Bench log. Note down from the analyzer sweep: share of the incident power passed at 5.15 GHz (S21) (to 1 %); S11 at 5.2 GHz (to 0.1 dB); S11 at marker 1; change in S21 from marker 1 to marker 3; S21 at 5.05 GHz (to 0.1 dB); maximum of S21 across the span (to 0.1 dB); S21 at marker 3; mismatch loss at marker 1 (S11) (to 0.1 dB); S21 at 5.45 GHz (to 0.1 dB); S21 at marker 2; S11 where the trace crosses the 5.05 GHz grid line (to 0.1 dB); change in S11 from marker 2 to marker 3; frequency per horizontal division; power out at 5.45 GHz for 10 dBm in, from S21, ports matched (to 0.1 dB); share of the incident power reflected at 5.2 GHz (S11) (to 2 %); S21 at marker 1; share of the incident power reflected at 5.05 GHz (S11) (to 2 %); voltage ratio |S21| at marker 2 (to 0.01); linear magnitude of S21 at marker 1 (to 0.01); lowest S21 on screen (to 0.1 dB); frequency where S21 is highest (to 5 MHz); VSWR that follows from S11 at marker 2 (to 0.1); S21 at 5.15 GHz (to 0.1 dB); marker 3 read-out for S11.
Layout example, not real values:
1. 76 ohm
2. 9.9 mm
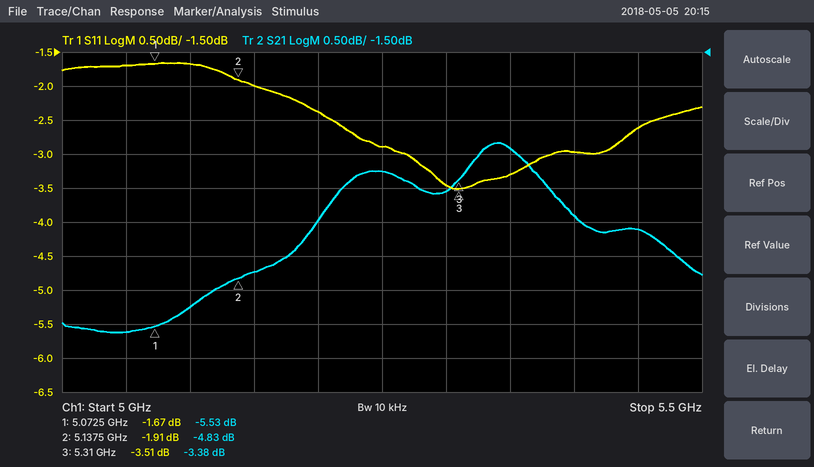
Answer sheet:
1. 34 %
2. -2.4 dB
3. -1.67 dB
4. 2.15 dB
5. -5.6 dB
6. -2.8 dB
7. -3.38 dB
8. 5.0 dB
9. -4.1 dB
10. -4.83 dB
11. -1.7 dB
12. -1.60 dB
13. 50 MHz
14. 5.9 dBm
15. 58 %
16. -5.53 dB
17. 68 %
18. 0.57
19. 0.53
20. -5.6 dB
21. 5.340 GHz
22. 9.1
23. -4.7 dB
24. -3.51 dB
